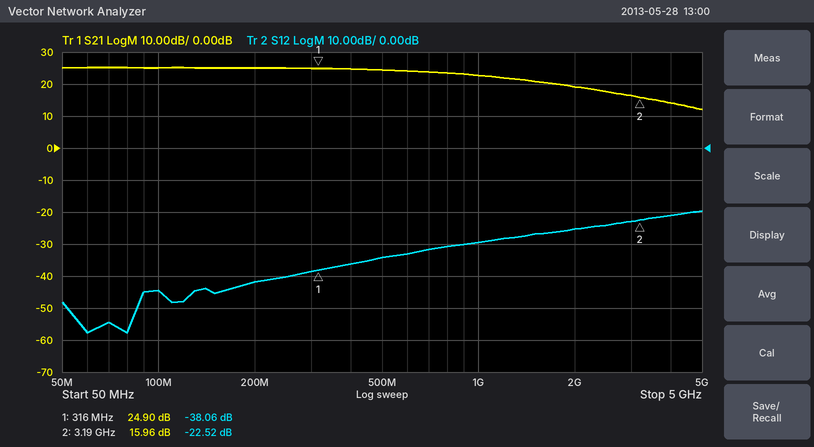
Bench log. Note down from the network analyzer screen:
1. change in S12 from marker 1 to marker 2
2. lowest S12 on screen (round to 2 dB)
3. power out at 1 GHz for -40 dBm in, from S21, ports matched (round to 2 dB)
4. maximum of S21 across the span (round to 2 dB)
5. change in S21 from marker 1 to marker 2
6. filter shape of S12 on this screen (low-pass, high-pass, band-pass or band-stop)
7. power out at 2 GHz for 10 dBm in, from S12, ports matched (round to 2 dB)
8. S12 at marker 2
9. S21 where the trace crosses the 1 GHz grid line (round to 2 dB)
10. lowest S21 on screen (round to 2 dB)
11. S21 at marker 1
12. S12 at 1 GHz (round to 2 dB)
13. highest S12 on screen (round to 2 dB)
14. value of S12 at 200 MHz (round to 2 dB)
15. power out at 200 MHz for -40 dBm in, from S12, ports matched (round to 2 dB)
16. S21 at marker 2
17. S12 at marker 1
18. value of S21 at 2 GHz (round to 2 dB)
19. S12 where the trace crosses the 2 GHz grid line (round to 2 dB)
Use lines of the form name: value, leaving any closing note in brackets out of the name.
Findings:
change in S12 from marker 1 to marker 2: 15.54 dB
lowest S12 on screen: -58 dB
power out at 1 GHz for -40 dBm in, from S21, ports matched: -18 dBm
maximum of S21 across the span: 26 dB
change in S21 from marker 1 to marker 2: -8.94 dB
filter shape of S12 on this screen: high-pass
power out at 2 GHz for 10 dBm in, from S12, ports matched: -16 dBm
S12 at marker 2: -22.52 dB
S21 where the trace crosses the 1 GHz grid line: 22 dB
lowest S21 on screen: 12 dB
S21 at marker 1: 24.90 dB
S12 at 1 GHz: -30 dB
highest S12 on screen: -20 dB
value of S12 at 200 MHz: -42 dB
power out at 200 MHz for -40 dBm in, from S12, ports matched: -82 dBm
S21 at marker 2: 15.96 dB
S12 at marker 1: -38.06 dB
value of S21 at 2 GHz: 20 dB
S12 where the trace crosses the 2 GHz grid line: -26 dB
